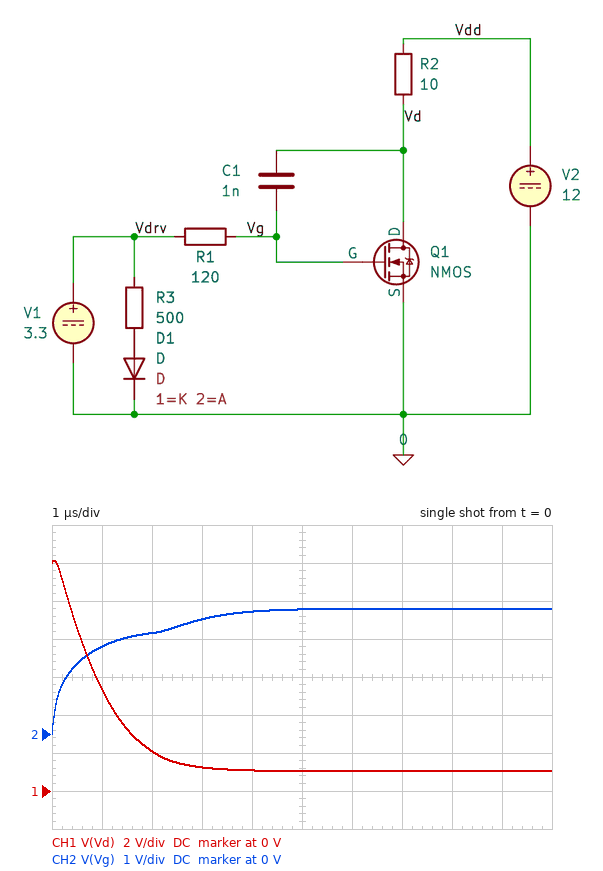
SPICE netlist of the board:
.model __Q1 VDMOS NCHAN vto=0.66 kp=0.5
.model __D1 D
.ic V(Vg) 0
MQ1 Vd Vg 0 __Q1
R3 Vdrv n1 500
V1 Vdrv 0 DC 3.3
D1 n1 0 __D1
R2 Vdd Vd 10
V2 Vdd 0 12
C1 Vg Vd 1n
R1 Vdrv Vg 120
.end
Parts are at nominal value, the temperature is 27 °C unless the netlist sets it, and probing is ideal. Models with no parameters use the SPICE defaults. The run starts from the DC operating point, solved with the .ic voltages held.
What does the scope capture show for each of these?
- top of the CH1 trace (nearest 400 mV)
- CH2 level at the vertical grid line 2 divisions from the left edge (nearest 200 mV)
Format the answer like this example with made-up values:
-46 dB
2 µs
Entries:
12.0 V
2.6 V
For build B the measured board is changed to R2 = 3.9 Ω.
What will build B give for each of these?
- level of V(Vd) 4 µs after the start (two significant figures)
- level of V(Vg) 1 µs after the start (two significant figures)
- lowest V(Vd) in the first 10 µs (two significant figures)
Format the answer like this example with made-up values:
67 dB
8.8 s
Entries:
5.4 V
2.7 V
5.2 V
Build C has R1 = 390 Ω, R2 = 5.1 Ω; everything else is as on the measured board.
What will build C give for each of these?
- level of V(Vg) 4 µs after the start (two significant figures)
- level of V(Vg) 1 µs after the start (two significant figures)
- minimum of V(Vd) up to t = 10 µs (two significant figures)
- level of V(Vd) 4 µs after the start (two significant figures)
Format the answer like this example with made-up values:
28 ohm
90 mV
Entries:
2.7 V
1.7 V
4.1 V
6.5 V
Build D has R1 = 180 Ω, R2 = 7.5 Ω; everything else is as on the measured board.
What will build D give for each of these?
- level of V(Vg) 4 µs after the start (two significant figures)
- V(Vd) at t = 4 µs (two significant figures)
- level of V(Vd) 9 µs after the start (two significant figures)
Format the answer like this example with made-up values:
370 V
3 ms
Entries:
2.9 V
2.4 V
1.5 V
